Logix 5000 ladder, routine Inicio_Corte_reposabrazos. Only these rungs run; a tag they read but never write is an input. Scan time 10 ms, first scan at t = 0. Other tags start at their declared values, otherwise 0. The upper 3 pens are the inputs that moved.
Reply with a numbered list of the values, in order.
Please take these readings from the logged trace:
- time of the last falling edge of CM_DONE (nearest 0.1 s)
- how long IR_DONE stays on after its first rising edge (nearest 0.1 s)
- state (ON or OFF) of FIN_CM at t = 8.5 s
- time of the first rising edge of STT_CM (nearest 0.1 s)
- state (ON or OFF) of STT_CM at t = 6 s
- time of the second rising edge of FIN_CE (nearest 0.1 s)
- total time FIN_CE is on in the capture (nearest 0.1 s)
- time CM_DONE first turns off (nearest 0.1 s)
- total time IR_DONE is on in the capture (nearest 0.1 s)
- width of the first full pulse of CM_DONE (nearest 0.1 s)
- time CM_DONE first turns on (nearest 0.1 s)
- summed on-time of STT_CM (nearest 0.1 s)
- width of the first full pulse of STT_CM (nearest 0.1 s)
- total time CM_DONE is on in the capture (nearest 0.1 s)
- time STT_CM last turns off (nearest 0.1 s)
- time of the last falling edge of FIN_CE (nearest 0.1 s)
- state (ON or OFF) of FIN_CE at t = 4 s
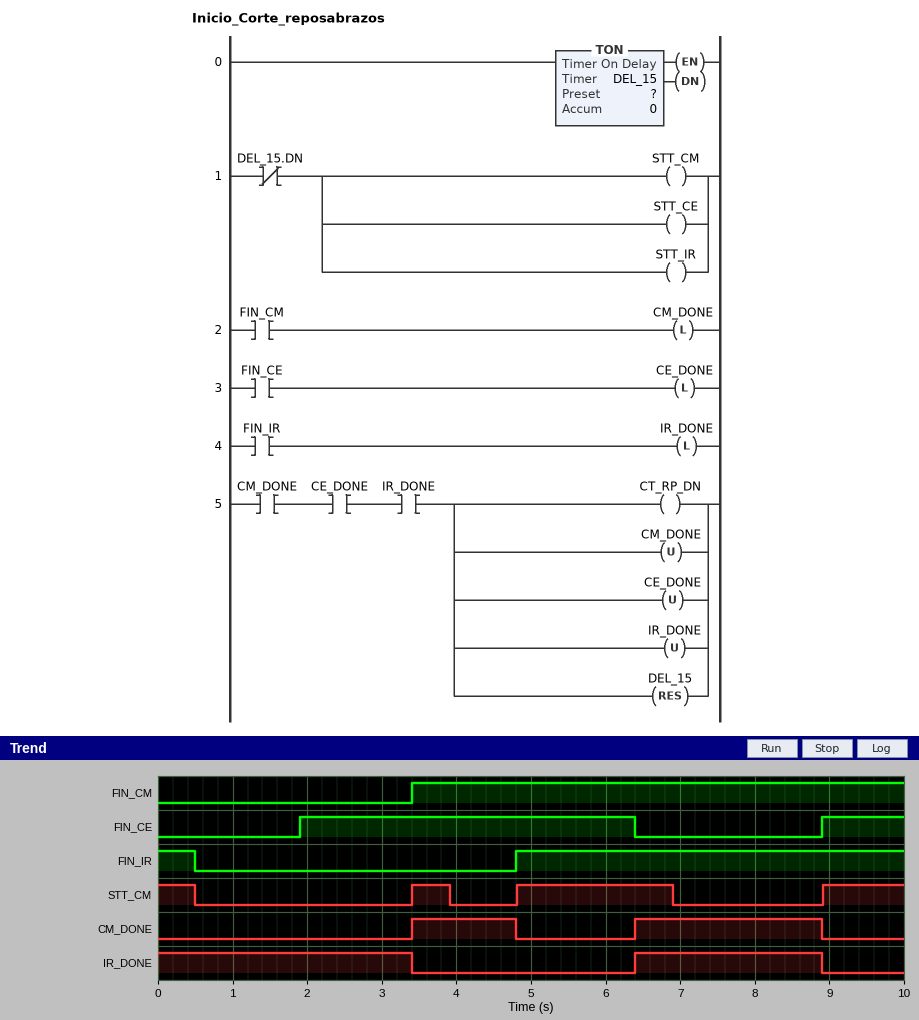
1. 8.9 s
2. 2.5 s
3. ON
4. 3.4 s
5. ON
6. 8.9 s
7. 5.6 s
8. 4.8 s
9. 5.9 s
10. 1.4 s
11. 3.4 s
12. 4.2 s
13. 0.5 s
14. 3.9 s
15. 6.9 s
16. 6.4 s
17. ON
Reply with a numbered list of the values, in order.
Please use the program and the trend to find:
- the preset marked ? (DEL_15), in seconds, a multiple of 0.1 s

1. 0.5 s
